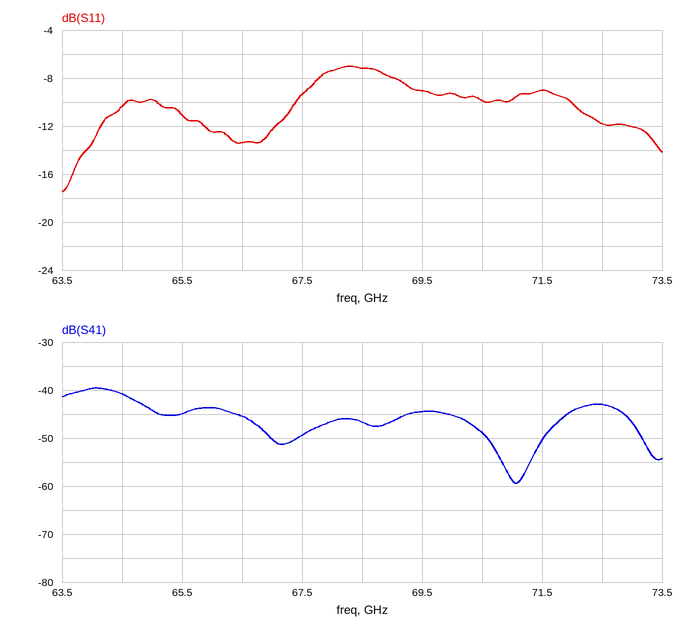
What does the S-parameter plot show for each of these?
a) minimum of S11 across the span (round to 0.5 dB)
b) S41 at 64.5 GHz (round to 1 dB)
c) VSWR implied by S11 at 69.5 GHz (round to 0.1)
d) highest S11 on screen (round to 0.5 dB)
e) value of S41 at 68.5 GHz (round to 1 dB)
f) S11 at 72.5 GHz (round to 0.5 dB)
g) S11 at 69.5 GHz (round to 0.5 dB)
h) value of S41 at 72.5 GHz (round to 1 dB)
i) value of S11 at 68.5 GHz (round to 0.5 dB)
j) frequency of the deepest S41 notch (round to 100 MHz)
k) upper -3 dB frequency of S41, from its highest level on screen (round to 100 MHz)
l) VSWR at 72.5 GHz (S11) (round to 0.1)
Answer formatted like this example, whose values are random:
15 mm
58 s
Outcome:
-17.5 dB
-41 dB
2.1
-7.0 dB
-47 dB
-12.0 dB
-9.0 dB
-43 dB
-7.0 dB
71.1 GHz
64.8 GHz
1.7
